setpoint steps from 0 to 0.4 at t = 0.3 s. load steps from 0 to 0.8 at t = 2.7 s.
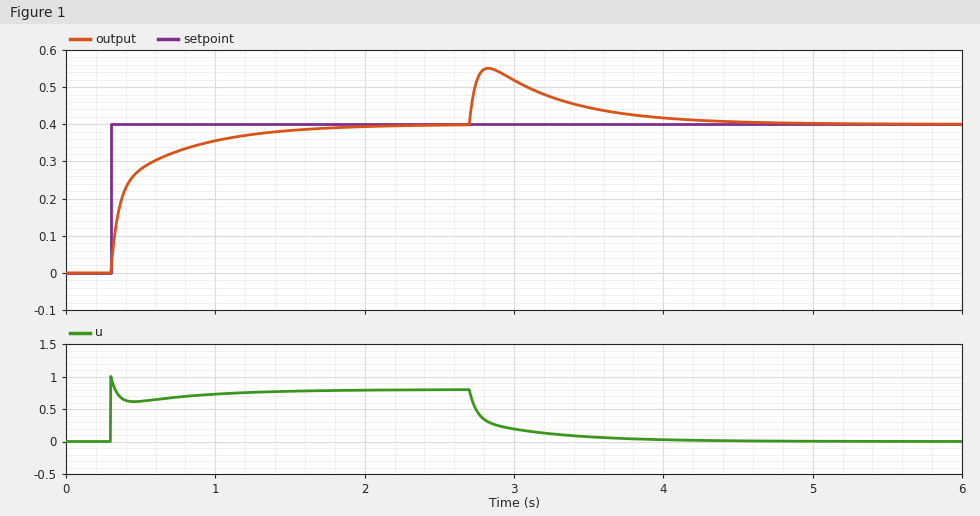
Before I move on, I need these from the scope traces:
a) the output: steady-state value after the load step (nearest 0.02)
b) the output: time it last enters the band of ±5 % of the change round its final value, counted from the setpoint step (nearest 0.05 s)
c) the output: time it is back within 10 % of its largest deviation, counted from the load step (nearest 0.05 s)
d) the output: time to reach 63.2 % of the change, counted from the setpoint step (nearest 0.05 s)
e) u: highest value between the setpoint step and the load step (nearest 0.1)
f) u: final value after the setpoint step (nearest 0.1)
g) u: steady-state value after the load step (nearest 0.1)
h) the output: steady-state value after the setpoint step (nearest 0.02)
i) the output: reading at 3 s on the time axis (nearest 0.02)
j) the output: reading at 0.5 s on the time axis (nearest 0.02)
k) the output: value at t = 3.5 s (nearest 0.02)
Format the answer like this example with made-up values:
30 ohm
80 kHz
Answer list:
0.40
1.10 s
1.35 s
0.15 s
1.0
0.8
0.0
0.40
0.52
0.28
0.44
